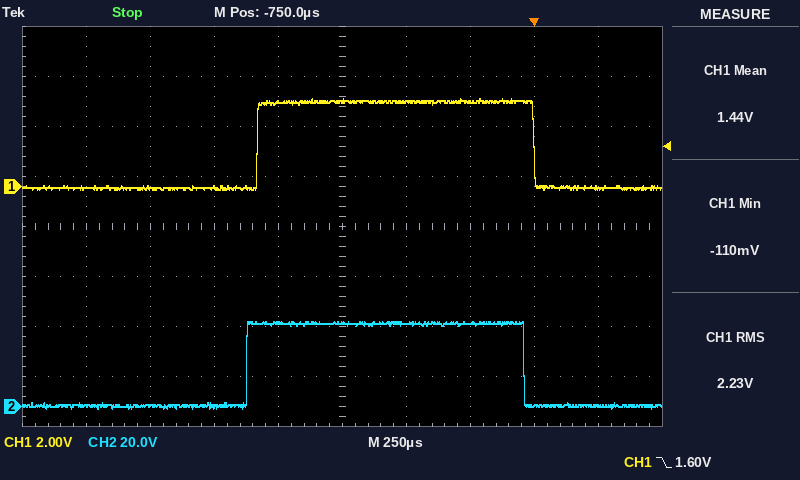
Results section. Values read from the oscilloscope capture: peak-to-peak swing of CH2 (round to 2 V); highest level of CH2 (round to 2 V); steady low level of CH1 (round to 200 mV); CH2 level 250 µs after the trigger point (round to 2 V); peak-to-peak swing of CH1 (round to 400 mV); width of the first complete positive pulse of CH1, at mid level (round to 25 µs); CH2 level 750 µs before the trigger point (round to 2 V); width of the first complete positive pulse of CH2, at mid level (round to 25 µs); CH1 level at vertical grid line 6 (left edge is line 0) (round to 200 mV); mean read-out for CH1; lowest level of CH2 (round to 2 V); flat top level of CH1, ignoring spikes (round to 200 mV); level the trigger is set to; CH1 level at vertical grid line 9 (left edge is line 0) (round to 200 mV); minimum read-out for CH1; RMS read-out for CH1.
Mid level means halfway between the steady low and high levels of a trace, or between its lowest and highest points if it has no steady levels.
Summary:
34 V
34 V
0.0 V
0 V
3.6 V
1.075 ms
34 V
1.075 ms
3.4 V
1.44 V
0 V
3.4 V
1.60 V
0.0 V
-110 mV
2.23 V
